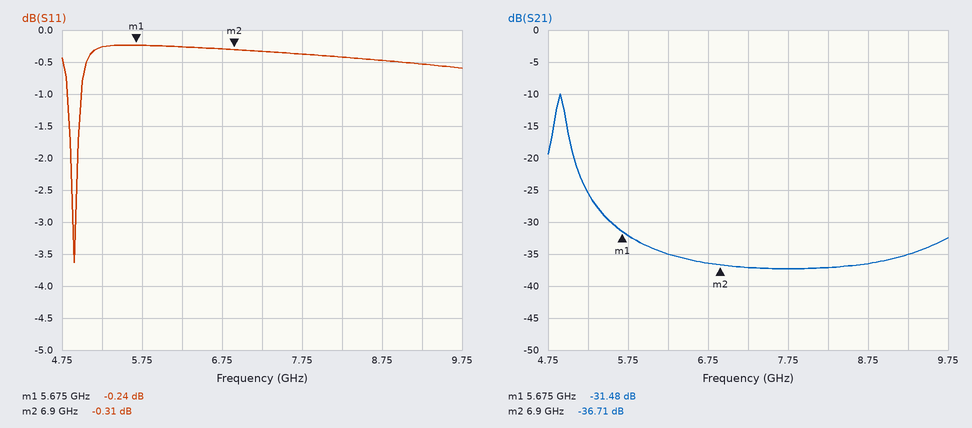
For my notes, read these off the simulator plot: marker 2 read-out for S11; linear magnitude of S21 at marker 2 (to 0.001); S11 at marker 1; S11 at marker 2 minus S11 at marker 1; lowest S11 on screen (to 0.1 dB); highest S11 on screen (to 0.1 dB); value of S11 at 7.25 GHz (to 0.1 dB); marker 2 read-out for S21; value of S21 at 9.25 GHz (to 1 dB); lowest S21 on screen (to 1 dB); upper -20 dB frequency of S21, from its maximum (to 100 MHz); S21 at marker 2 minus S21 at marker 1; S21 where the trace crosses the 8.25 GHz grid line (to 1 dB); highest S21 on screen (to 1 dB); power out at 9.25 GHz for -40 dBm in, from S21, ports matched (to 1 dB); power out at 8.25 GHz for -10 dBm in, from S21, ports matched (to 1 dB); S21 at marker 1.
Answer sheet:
-0.31 dB
0.015
-0.24 dB
-0.07 dB
-3.6 dB
-0.2 dB
-0.3 dB
-36.71 dB
-35 dB
-37 dB
5.5 GHz
-5.23 dB
-37 dB
-10 dB
-75 dBm
-47 dBm
-31.48 dB
